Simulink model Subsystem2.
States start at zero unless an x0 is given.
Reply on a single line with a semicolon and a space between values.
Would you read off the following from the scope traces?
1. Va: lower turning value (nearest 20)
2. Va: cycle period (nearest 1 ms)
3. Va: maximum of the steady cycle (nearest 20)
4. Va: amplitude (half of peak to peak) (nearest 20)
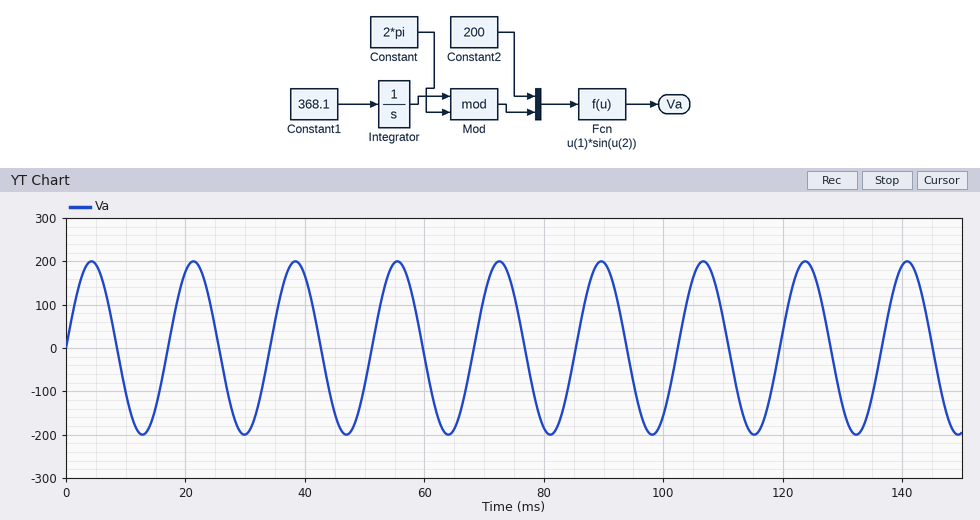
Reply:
-200; 17 ms; 200; 200
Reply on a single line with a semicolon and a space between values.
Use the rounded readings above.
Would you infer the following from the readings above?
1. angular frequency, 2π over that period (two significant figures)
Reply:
0.37 rad/ms
